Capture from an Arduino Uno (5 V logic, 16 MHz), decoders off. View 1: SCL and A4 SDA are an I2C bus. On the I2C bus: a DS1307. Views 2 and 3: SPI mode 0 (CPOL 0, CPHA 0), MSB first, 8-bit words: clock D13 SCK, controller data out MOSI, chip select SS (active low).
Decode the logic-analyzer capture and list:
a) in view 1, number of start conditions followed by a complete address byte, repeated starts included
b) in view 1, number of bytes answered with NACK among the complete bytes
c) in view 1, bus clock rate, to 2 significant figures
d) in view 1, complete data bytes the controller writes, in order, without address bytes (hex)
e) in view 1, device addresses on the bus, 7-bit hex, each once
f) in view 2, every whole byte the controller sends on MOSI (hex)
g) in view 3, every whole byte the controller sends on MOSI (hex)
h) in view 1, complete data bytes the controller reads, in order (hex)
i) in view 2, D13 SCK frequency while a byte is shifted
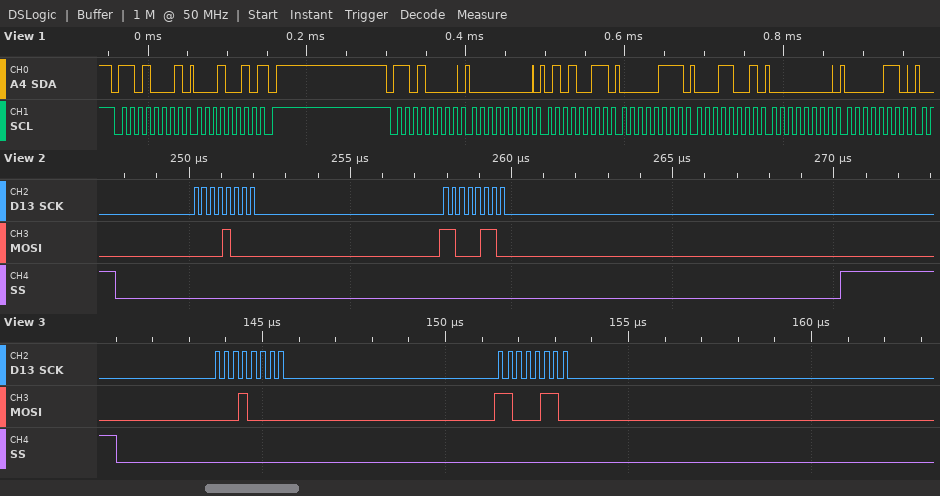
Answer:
2
1
100 kHz
00 53 07 19 00 06
0x68
08 C6
0x10 0xC6
12
4 MHz
